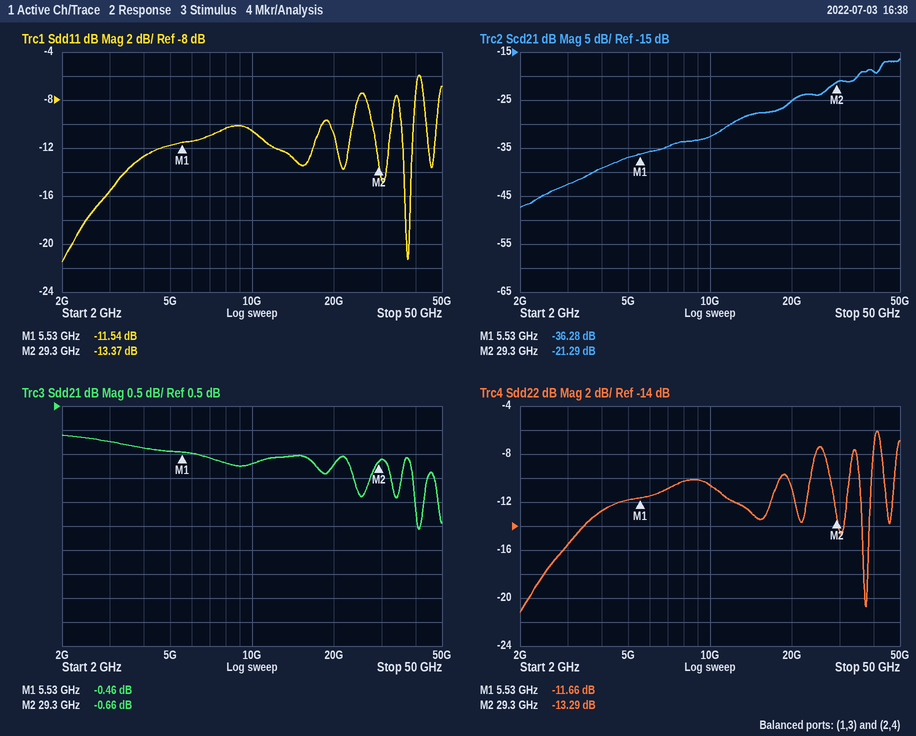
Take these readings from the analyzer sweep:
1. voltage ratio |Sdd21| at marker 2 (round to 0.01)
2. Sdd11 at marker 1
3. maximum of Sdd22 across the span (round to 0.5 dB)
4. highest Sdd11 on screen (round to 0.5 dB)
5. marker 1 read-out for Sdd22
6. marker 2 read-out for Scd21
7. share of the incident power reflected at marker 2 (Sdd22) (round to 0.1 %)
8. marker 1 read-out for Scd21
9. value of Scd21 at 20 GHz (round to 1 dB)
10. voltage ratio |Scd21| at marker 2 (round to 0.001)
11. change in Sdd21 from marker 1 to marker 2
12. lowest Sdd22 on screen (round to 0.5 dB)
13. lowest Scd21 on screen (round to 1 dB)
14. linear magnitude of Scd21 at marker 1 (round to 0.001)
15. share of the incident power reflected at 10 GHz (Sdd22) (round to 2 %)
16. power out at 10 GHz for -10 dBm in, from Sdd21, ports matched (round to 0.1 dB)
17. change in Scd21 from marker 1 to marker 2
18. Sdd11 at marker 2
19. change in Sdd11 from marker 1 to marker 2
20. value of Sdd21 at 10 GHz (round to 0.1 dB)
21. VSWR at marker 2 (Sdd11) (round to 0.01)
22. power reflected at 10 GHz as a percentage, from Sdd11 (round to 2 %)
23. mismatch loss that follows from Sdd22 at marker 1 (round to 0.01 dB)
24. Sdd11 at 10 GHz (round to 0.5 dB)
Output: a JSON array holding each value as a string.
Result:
["0.93", "-11.54 dB", "-6.0 dB", "-6.0 dB", "-11.66 dB", "-21.29 dB", "4.7 %", "-36.28 dB", "-25 dB", "0.086", "-0.20 dB", "-21.0 dB", "-47 dB", "0.015", "8 %", "-10.7 dBm", "14.99 dB", "-13.37 dB", "-1.83 dB", "-0.7 dB", "1.55", "8 %", "0.31 dB", "-10.5 dB"]
